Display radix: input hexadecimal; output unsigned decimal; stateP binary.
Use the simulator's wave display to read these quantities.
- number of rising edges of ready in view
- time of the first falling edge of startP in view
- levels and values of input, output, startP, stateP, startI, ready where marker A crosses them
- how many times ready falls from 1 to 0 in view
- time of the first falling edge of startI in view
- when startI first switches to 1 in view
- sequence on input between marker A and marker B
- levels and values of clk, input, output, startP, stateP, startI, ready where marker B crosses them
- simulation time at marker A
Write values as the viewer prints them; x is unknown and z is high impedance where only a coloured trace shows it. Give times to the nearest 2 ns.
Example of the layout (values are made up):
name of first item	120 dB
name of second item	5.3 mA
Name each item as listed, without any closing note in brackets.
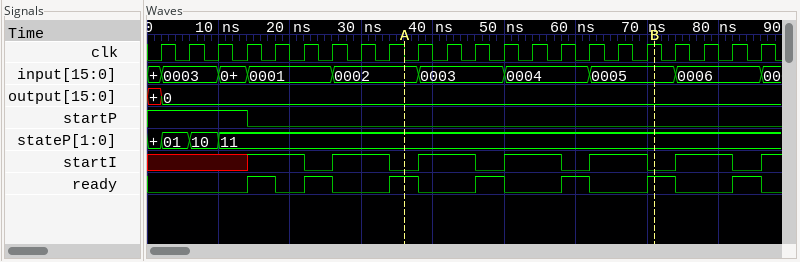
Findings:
number of rising edges of ready in view	7
time of the first falling edge of startP in view	14 ns
levels and values of input, output, startP, stateP, startI, ready where marker A crosses them	input=0002, output=0, startP=0, stateP=11, startI=0, ready=1
how many times ready falls from 1 to 0 in view	7
time of the first falling edge of startI in view	22 ns
when startI first switches to 1 in view	14 ns
sequence on input between marker A and marker B	0002, 0003, 0004, 0005
levels and values of clk, input, output, startP, stateP, startI, ready where marker B crosses them	clk=1, input=0005, output=0, startP=0, stateP=11, startI=0, ready=1
simulation time at marker A	36 ns
